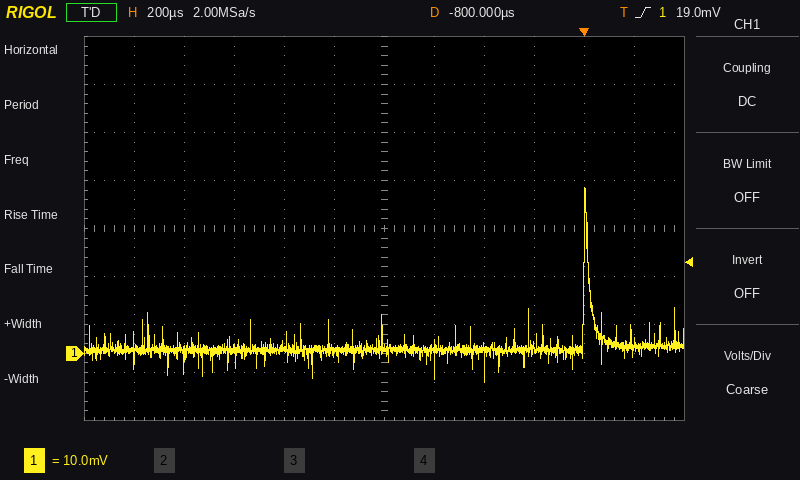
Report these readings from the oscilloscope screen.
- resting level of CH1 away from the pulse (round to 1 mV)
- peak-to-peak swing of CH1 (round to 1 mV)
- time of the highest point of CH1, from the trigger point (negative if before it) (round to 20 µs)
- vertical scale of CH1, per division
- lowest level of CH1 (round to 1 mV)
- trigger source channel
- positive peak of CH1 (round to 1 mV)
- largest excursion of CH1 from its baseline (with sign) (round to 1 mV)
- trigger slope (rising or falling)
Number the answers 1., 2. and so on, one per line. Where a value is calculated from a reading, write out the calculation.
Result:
1. 1 mV
2. 35 mV − (-6 mV) = 41 mV
3. 0 µs
4. 10 mV
5. -6 mV
6. CH1
7. 35 mV
8. 35 mV − (1 mV) = +34 mV
9. rising
